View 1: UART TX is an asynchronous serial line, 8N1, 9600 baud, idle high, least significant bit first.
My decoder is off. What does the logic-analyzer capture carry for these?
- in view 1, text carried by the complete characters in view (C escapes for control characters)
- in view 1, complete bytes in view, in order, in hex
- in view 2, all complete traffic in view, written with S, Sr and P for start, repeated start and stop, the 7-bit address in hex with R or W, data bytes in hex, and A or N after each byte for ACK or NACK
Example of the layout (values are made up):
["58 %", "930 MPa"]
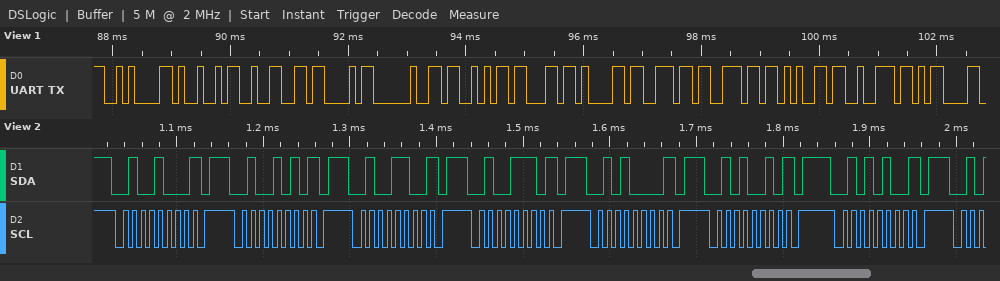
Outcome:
["\"\\nI2C Scanner\\r\"", "0x0A 0x49 0x32 0x43 0x20 0x53 0x63 0x61 0x6E 0x6E 0x65 0x72 0x0D", "S 24W N P S 25W N P S 26W N P S 27W N P S 28W N P S 29W N P S 2AW N P"]
